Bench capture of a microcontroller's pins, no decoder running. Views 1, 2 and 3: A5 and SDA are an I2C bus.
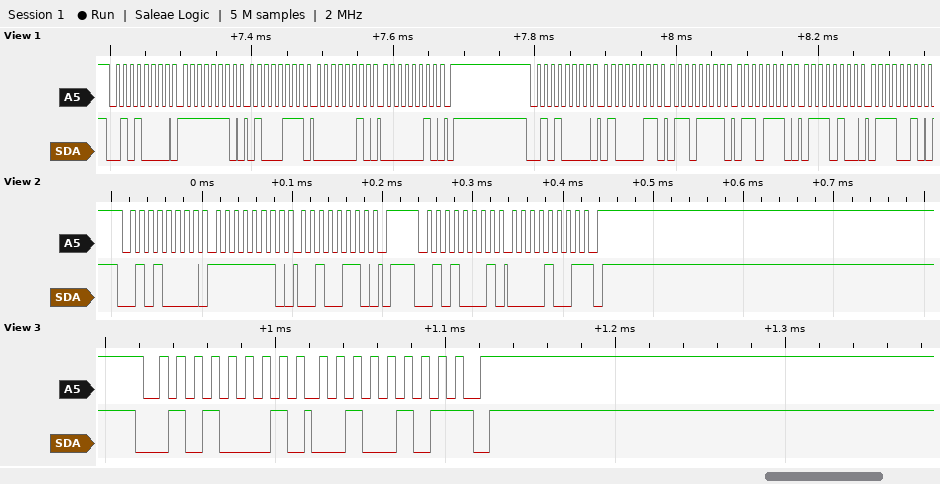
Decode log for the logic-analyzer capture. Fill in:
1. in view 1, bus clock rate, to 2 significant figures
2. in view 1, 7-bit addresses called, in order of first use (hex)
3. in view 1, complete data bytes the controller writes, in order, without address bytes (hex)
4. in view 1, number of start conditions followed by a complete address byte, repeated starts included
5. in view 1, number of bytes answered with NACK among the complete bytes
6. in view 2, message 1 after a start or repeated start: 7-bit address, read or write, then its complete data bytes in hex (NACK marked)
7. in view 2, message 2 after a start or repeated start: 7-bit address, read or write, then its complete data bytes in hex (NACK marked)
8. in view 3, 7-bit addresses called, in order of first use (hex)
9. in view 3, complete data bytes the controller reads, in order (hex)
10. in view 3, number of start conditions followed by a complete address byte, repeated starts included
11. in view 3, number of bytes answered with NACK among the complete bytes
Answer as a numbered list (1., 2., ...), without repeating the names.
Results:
1. 100 kHz
2. 0x28
3. FE 47 02 02 43 6F 6E 74 72
4. 2
5. 0
6. 0x28 write: FE 26
7. 0x28 read: 09 NACK
8. 0x28
9. 25
10. 1
11. 1
